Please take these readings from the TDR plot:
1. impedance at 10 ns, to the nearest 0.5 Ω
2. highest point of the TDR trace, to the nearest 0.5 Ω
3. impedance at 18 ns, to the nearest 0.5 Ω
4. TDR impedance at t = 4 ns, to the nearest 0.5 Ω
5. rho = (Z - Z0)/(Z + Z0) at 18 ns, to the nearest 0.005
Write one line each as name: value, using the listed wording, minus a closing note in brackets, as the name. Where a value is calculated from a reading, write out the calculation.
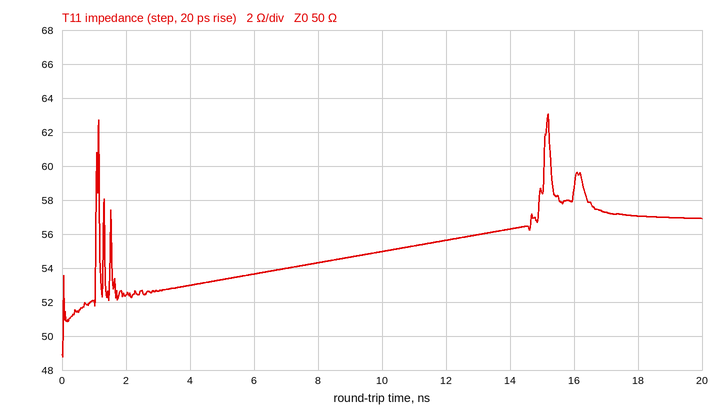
impedance at 10 ns, to the nearest 0.5 Ω: 55.0 Ω
highest point of the TDR trace, to the nearest 0.5 Ω: 63.0 Ω
impedance at 18 ns, to the nearest 0.5 Ω: 57.0 Ω
TDR impedance at t = 4 ns, to the nearest 0.5 Ω: 53.0 Ω
rho = (Z - Z0)/(Z + Z0) at 18 ns, to the nearest 0.005: (57 − 50)/(57 + 50) ≈ +0.065
